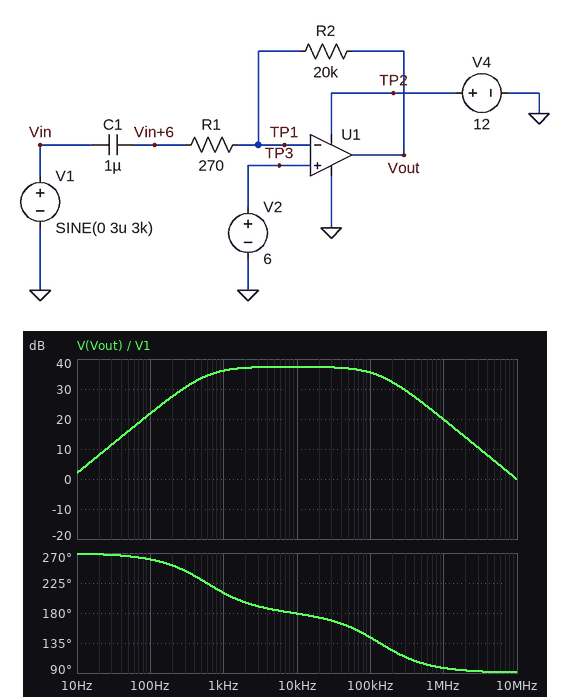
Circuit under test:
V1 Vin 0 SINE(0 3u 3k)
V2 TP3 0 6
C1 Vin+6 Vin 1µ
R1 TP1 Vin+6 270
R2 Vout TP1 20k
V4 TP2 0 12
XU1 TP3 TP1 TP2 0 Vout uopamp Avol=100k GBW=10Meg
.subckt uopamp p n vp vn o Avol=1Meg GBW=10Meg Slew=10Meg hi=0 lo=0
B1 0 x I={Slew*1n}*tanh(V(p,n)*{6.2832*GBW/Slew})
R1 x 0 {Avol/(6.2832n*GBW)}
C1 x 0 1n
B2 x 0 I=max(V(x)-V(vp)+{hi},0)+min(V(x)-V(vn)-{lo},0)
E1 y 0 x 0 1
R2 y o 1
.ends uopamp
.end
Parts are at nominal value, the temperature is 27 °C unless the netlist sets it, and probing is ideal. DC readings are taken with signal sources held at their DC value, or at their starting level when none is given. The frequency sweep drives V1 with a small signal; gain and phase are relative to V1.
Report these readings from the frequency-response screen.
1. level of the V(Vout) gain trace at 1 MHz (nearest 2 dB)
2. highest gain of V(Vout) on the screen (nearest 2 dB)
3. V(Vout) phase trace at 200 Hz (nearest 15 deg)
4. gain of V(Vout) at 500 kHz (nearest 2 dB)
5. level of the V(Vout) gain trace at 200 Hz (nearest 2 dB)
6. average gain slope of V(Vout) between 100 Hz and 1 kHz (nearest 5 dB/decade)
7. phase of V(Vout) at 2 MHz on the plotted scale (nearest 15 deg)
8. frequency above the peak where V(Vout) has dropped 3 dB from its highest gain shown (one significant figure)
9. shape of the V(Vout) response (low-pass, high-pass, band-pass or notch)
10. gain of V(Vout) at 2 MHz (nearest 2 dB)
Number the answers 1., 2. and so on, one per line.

1. 20 dB
2. 38 dB
3. 255 deg
4. 26 dB
5. 28 dB
6. 15 dB/decade
7. 90 deg
8. 100 kHz
9. band-pass
10. 14 dB
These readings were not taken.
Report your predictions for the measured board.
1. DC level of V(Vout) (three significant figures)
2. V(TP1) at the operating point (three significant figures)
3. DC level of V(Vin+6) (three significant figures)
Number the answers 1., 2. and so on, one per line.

1. 6.00 V
2. 6.00 V
3. 6.00 V
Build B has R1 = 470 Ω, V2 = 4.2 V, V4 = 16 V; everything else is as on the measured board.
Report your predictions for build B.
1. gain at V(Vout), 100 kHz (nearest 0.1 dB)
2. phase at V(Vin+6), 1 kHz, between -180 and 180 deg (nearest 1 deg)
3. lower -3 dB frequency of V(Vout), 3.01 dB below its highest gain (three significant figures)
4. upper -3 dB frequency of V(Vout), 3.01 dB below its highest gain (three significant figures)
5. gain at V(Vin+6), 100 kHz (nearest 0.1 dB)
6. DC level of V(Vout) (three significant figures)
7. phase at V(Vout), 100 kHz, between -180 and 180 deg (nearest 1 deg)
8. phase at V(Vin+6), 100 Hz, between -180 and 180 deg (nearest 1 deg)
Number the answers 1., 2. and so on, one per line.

1. 31.8 dB
2. 19 deg
3. 338 Hz
4. 230 kHz
5. 0 dB
6. 4.20 V
7. 157 deg
8. 74 deg
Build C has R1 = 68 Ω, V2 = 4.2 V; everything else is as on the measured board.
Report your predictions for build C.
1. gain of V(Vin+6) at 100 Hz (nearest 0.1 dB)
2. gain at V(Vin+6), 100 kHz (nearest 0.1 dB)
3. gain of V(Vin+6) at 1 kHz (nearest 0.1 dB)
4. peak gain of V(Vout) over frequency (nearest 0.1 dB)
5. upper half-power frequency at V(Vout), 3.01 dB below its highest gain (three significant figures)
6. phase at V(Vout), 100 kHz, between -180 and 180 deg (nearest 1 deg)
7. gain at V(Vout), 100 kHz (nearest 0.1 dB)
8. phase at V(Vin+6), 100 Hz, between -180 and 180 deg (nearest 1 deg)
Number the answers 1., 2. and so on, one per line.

1. -27.4 dB
2. 0.1 dB
3. -8.0 dB
4. 49.3 dB
5. 36.2 kHz
6. 109 deg
7. 39.6 dB
8. 88 deg
